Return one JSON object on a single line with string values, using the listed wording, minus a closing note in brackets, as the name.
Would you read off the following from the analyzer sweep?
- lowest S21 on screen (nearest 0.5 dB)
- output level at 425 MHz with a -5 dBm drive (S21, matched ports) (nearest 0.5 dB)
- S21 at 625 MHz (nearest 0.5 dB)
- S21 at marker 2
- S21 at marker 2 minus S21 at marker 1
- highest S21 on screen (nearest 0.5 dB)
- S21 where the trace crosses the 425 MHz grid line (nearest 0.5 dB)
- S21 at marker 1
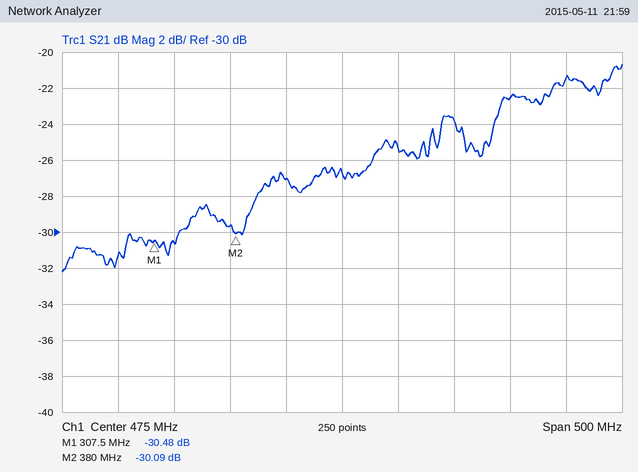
{"lowest S21 on screen": "-32.0 dB", "output level at 425 MHz with a -5 dBm drive (S21, matched ports)": "-32.0 dBm", "S21 at 625 MHz": "-22.5 dB", "S21 at marker 2": "-30.09 dB", "S21 at marker 2 minus S21 at marker 1": "0.39 dB", "highest S21 on screen": "-20.5 dB", "S21 where the trace crosses the 425 MHz grid line": "-27.0 dB", "S21 at marker 1": "-30.48 dB"}
